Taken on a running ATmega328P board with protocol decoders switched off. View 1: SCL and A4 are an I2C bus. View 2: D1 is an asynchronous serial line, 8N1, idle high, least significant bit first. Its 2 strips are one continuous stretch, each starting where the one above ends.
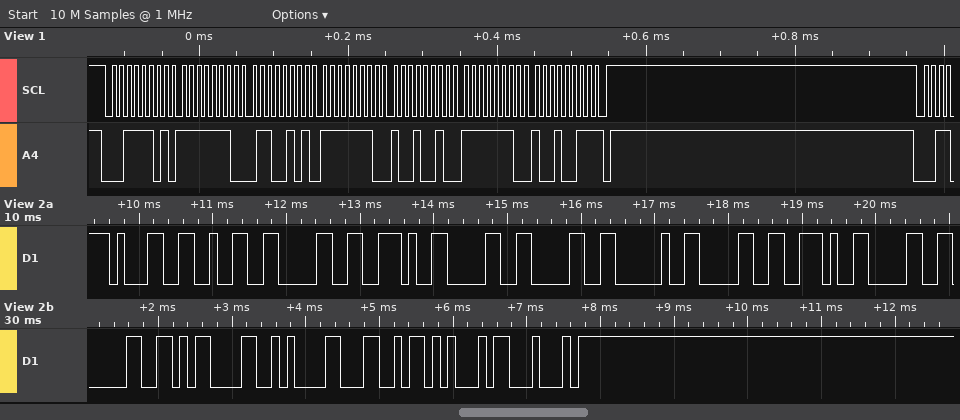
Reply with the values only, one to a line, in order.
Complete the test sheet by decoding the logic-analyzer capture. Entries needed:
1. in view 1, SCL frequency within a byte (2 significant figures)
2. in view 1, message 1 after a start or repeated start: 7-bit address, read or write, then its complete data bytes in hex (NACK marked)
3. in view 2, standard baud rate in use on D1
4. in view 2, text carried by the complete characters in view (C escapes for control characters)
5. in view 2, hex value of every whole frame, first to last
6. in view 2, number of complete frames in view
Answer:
100 kHz
0x1E read: FE 65 FE 92 FE 93 NACK
9600 baud
"120.00 0.00\r\nLED"
31 32 30 2E 30 30 20 30 2E 30 30 0D 0A 4C 45 44
16
